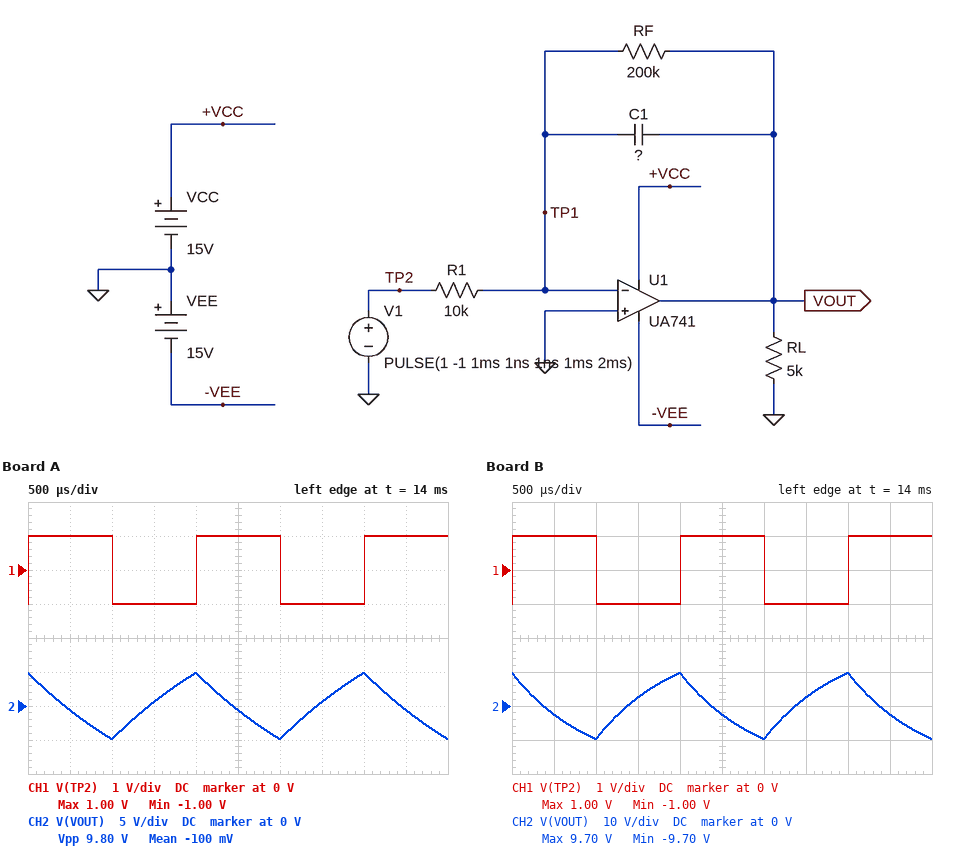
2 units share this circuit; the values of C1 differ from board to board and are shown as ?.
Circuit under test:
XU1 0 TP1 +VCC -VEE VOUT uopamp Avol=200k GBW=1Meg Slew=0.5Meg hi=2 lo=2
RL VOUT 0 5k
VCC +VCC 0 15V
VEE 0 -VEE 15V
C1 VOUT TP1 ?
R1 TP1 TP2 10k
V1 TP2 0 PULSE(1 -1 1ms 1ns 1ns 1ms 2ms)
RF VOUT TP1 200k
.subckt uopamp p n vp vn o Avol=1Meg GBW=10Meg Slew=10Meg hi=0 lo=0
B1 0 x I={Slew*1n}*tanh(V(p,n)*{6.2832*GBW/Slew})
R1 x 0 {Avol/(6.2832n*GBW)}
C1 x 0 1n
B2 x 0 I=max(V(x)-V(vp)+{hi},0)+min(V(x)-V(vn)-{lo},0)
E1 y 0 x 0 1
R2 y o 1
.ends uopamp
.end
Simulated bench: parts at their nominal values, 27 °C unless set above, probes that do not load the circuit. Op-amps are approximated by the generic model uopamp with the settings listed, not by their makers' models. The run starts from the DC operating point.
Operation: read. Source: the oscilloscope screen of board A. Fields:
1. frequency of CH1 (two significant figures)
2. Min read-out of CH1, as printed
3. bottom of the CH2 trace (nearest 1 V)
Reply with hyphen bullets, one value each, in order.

- 500 Hz
- -1.00 V
- -5 V
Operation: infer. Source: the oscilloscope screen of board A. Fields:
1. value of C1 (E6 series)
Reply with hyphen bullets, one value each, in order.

- 10 nF
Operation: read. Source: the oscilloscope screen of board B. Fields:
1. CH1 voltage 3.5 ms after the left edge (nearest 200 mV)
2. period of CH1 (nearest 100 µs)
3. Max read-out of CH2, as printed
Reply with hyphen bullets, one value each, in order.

- -1.0 V
- 2.0 ms
- 9.70 V
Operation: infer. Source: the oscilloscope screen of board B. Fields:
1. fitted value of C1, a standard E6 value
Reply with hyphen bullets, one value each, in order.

- 4.7 nF
